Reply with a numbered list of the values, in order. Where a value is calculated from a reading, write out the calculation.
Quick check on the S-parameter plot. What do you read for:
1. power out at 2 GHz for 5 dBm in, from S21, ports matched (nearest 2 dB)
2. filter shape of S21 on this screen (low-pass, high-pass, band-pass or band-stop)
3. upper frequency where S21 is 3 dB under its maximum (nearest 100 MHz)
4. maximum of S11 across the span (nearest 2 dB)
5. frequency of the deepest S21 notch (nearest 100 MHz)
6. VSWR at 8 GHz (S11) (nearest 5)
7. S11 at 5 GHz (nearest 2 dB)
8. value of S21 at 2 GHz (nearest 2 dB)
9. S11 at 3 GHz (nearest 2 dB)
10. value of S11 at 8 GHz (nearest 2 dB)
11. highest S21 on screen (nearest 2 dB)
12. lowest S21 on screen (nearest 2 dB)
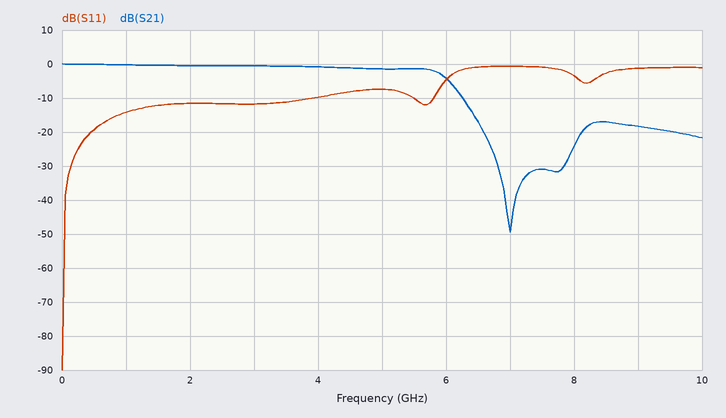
1. 5 dBm + (0 dB) = 4 dBm
2. low-pass
3. 5.9 GHz
4. 0 dB
5. 7.0 GHz
6. |Γ| = 10^(-4/20) = 0.6310; VSWR = (1 + 0.6310)/(1 − 0.6310) ≈ 4.42, so 5 to the nearest 5
7. -8 dB
8. 0 dB
9. -12 dB
10. -4 dB
11. 0 dB
12. -50 dB
